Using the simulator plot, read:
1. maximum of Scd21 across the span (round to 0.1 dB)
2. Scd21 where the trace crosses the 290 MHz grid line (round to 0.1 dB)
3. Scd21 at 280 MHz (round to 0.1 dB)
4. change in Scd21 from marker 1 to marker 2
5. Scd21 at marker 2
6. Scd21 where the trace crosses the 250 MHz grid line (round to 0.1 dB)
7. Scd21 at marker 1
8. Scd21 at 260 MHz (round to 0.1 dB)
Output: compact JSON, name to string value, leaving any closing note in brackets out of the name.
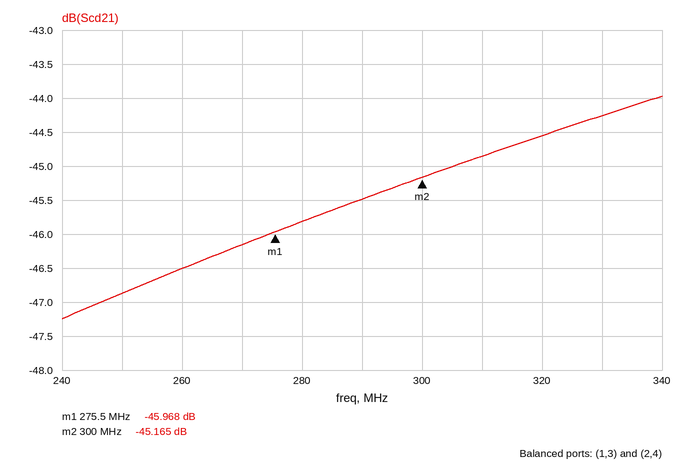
{"maximum of Scd21 across the span": "-44.0 dB", "Scd21 where the trace crosses the 290 MHz grid line": "-45.5 dB", "Scd21 at 280 MHz": "-45.8 dB", "change in Scd21 from marker 1 to marker 2": "0.803 dB", "Scd21 at marker 2": "-45.165 dB", "Scd21 where the trace crosses the 250 MHz grid line": "-46.9 dB", "Scd21 at marker 1": "-45.968 dB", "Scd21 at 260 MHz": "-46.5 dB"}
